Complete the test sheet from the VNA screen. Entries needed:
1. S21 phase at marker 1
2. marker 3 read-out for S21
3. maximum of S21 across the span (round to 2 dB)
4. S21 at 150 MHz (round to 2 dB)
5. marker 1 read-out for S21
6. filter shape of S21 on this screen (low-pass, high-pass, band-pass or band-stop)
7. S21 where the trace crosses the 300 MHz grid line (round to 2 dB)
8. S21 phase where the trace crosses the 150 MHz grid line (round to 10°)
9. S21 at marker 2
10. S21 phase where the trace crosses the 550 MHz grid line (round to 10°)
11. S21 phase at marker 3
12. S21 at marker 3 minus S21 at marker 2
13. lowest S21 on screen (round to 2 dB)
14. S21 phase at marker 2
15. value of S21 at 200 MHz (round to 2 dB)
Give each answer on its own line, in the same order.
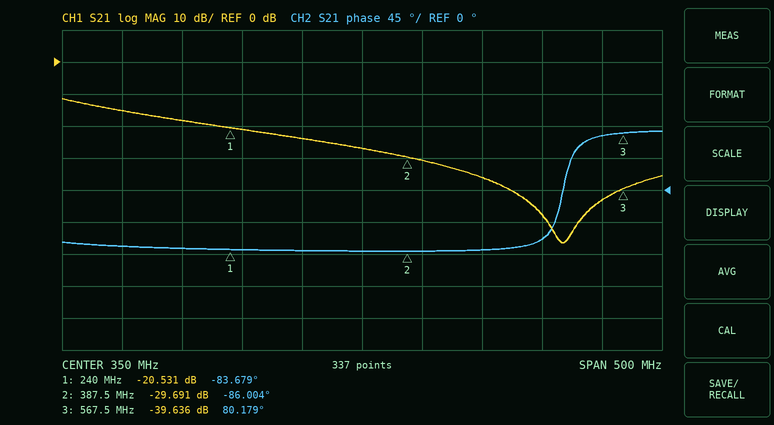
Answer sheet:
-83.679°
-39.636 dB
-12 dB
-16 dB
-20.531 dB
low-pass
-24 dB
-80°
-29.691 dB
80°
80.179°
-9.945 dB
-56 dB
-86.004°
-18 dB
